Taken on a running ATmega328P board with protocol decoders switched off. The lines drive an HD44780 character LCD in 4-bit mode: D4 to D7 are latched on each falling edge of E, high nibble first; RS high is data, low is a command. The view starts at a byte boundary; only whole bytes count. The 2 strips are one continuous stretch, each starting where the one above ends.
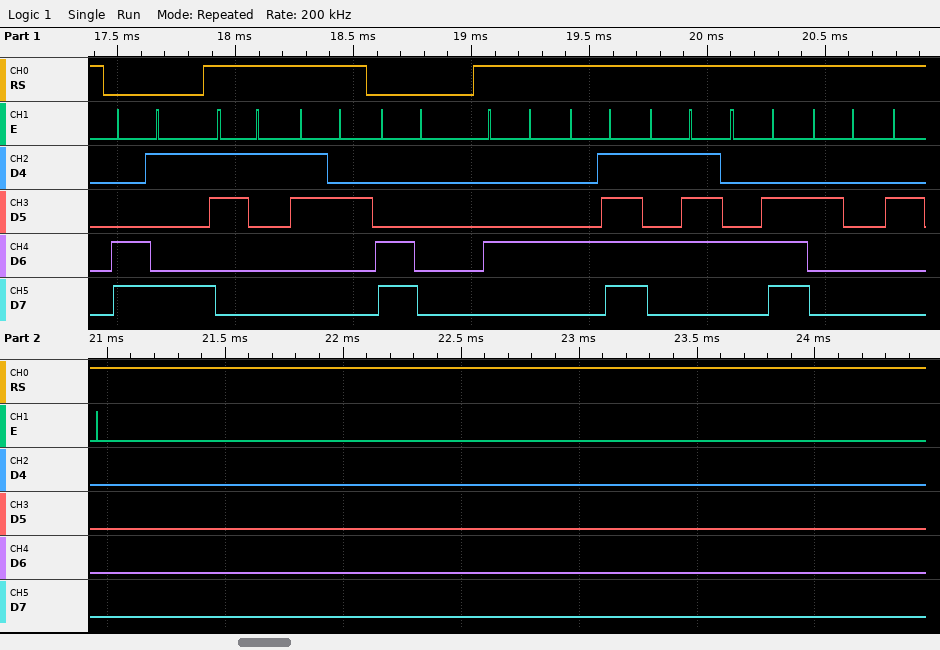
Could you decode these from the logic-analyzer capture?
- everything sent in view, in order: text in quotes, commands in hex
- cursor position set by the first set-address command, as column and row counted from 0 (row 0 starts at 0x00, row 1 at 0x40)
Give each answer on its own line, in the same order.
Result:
0xC9 "12" 0xC0 "DOWN  "
column 9, row 1
